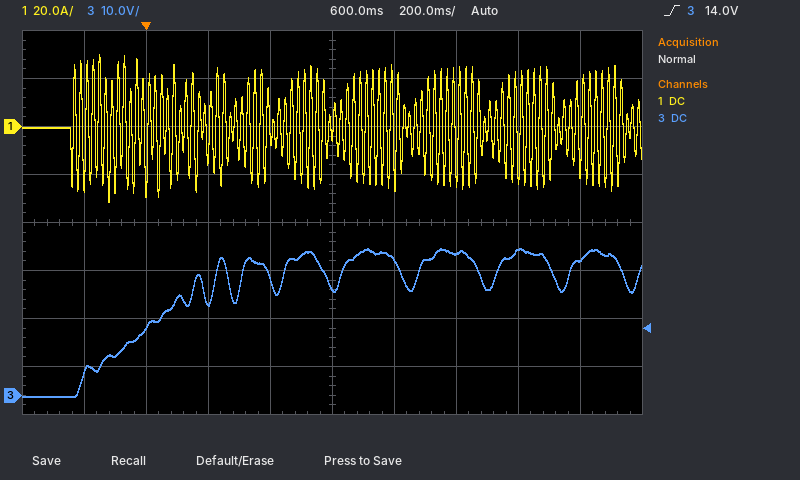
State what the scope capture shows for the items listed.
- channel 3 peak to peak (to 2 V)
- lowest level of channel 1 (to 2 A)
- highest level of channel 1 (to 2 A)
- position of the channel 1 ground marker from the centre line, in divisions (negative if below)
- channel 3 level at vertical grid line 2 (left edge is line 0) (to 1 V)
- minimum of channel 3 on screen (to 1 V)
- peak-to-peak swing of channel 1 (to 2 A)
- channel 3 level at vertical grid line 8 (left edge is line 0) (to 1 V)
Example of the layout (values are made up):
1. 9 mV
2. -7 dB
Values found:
1. 30 V
2. -32 A
3. 30 A
4. +2.0 div
5. 14 V
6. 0 V
7. 62 A
8. 30 V
